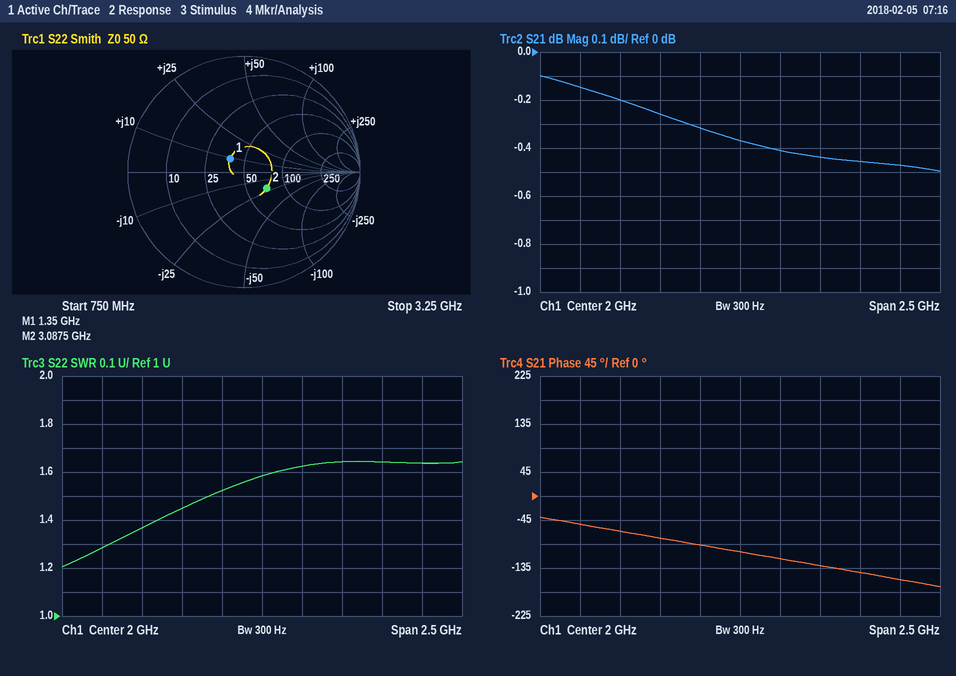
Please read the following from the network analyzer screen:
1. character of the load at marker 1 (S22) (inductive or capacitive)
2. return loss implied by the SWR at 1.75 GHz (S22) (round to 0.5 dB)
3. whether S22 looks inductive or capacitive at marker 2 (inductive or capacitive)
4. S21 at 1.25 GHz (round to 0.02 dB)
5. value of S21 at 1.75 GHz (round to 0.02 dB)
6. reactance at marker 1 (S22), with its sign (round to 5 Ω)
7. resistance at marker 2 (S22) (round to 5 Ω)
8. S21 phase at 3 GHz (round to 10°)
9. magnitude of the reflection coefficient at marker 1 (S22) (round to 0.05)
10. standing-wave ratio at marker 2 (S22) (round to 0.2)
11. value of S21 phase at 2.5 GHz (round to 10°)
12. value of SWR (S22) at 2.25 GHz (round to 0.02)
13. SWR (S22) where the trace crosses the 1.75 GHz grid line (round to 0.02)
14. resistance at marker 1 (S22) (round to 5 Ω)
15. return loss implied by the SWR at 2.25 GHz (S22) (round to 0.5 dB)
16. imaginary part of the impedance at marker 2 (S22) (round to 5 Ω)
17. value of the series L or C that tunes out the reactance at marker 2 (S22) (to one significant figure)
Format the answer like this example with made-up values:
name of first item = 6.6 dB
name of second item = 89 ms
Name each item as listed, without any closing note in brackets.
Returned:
character of the load at marker 1 (S22) = inductive
return loss implied by the SWR at 1.75 GHz (S22) = 13.5 dB
whether S22 looks inductive or capacitive at marker 2 = capacitive
S21 at 1.25 GHz = -0.20 dB
value of S21 at 1.75 GHz = -0.32 dB
reactance at marker 1 (S22), with its sign = +10 Ω
resistance at marker 2 (S22) = 70 Ω
S21 phase at 3 GHz = -160°
magnitude of the reflection coefficient at marker 1 (S22) = 0.15
standing-wave ratio at marker 2 (S22) = 1.6
value of S21 phase at 2.5 GHz = -130°
value of SWR (S22) at 2.25 GHz = 1.62
SWR (S22) where the trace crosses the 1.75 GHz grid line = 1.52
resistance at marker 1 (S22) = 40 Ω
return loss implied by the SWR at 2.25 GHz (S22) = 12.5 dB
imaginary part of the impedance at marker 2 (S22) = -20 Ω
value of the series L or C that tunes out the reactance at marker 2 (S22) = 1 nH
